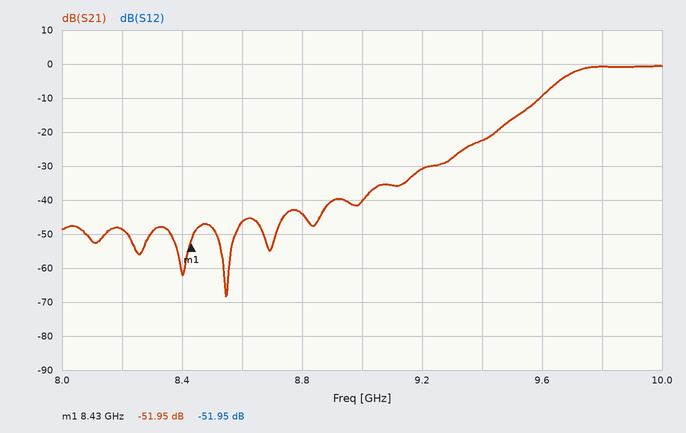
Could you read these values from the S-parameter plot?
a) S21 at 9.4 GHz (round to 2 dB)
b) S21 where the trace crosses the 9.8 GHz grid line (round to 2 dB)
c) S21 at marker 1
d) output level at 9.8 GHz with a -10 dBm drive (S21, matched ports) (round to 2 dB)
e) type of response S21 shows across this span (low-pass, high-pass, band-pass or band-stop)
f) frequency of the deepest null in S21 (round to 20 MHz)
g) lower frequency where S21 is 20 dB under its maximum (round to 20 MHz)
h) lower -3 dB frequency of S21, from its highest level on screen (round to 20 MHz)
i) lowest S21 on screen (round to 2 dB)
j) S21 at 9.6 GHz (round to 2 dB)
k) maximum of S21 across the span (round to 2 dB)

-22 dB
0 dB
-51.95 dB
-10 dBm
high-pass
8.54 GHz
9.44 GHz
9.68 GHz
-68 dB
-10 dB
0 dB
